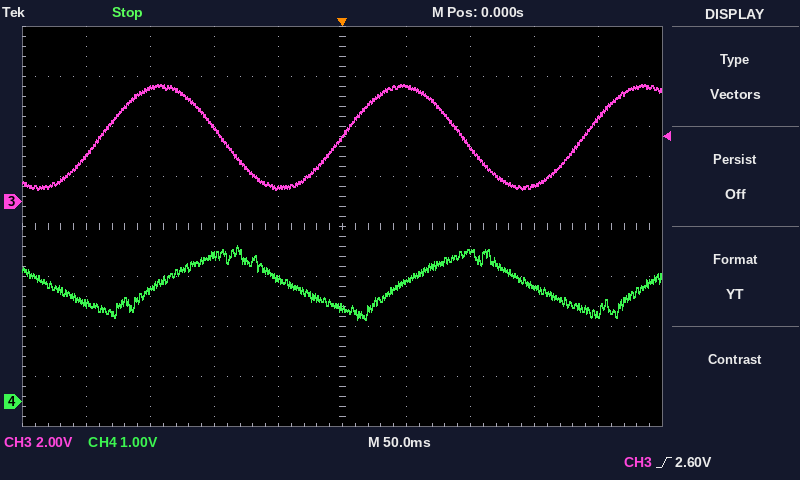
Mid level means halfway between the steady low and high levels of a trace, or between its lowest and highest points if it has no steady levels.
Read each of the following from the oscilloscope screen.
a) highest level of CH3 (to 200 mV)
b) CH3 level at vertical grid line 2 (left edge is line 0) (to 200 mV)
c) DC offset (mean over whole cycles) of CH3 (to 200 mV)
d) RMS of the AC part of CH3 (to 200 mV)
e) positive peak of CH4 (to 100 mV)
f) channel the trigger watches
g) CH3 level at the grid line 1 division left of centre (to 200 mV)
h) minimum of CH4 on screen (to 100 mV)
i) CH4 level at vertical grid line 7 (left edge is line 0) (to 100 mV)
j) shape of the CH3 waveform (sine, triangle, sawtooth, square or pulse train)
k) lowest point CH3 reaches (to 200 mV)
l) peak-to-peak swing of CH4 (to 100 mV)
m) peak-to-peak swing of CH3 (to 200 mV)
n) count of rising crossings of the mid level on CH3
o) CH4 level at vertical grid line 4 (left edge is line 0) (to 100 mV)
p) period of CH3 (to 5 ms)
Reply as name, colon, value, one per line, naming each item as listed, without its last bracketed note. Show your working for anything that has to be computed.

highest level of CH3: 4.6 V
CH3 level at vertical grid line 2 (left edge is line 0): 4.6 V
DC offset (mean over whole cycles) of CH3: (4.6 V + (400 mV)) / 2 ≈ 2.50 V, so 2.6 V to the nearest 200 mV
RMS of the AC part of CH3: 4.2 V / (2√2) ≈ 1.48 V, so 1.4 V to the nearest 200 mV
positive peak of CH4: 3.1 V
channel the trigger watches: CH3
CH3 level at the grid line 1 division left of centre: 600 mV
minimum of CH4 on screen: 1.6 V
CH4 level at vertical grid line 7 (left edge is line 0): 3.0 V
shape of the CH3 waveform: sine
lowest point CH3 reaches: 400 mV
peak-to-peak swing of CH4: 3.1 V − (1.6 V) = 1.5 V
peak-to-peak swing of CH3: 4.6 V − (400 mV) = 4.2 V
count of rising crossings of the mid level on CH3: 3
CH4 level at vertical grid line 4 (left edge is line 0): 2.4 V
period of CH3: 190 ms
